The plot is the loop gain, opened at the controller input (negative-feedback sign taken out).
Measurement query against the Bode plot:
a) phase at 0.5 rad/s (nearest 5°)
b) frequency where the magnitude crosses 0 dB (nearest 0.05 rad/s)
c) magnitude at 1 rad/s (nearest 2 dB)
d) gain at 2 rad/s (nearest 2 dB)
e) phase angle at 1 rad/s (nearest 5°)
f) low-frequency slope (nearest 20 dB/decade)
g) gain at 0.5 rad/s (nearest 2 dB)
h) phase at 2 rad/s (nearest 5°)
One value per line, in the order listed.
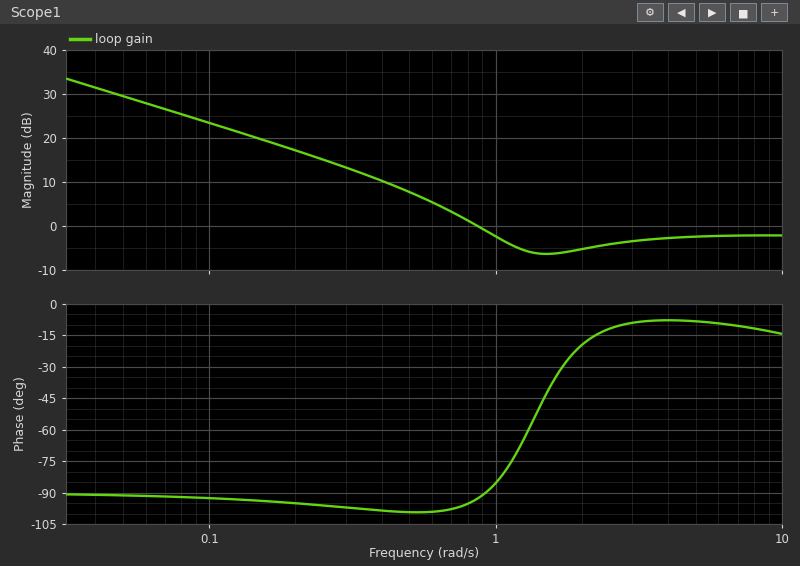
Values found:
-100°
0.85 rad/s
-2 dB
-6 dB
-85°
-20 dB/decade
8 dB
-20°
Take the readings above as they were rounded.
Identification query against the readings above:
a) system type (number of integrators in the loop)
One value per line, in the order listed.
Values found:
1
